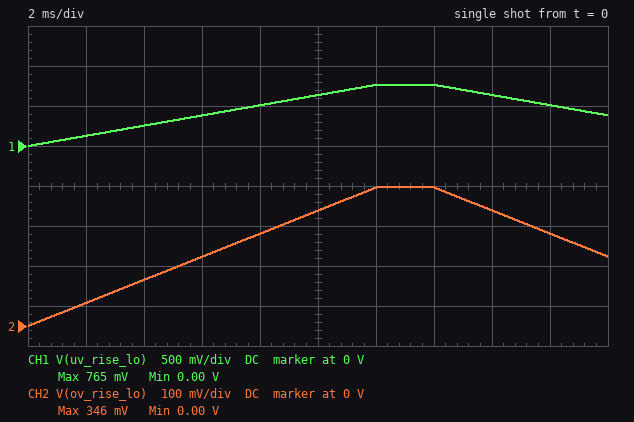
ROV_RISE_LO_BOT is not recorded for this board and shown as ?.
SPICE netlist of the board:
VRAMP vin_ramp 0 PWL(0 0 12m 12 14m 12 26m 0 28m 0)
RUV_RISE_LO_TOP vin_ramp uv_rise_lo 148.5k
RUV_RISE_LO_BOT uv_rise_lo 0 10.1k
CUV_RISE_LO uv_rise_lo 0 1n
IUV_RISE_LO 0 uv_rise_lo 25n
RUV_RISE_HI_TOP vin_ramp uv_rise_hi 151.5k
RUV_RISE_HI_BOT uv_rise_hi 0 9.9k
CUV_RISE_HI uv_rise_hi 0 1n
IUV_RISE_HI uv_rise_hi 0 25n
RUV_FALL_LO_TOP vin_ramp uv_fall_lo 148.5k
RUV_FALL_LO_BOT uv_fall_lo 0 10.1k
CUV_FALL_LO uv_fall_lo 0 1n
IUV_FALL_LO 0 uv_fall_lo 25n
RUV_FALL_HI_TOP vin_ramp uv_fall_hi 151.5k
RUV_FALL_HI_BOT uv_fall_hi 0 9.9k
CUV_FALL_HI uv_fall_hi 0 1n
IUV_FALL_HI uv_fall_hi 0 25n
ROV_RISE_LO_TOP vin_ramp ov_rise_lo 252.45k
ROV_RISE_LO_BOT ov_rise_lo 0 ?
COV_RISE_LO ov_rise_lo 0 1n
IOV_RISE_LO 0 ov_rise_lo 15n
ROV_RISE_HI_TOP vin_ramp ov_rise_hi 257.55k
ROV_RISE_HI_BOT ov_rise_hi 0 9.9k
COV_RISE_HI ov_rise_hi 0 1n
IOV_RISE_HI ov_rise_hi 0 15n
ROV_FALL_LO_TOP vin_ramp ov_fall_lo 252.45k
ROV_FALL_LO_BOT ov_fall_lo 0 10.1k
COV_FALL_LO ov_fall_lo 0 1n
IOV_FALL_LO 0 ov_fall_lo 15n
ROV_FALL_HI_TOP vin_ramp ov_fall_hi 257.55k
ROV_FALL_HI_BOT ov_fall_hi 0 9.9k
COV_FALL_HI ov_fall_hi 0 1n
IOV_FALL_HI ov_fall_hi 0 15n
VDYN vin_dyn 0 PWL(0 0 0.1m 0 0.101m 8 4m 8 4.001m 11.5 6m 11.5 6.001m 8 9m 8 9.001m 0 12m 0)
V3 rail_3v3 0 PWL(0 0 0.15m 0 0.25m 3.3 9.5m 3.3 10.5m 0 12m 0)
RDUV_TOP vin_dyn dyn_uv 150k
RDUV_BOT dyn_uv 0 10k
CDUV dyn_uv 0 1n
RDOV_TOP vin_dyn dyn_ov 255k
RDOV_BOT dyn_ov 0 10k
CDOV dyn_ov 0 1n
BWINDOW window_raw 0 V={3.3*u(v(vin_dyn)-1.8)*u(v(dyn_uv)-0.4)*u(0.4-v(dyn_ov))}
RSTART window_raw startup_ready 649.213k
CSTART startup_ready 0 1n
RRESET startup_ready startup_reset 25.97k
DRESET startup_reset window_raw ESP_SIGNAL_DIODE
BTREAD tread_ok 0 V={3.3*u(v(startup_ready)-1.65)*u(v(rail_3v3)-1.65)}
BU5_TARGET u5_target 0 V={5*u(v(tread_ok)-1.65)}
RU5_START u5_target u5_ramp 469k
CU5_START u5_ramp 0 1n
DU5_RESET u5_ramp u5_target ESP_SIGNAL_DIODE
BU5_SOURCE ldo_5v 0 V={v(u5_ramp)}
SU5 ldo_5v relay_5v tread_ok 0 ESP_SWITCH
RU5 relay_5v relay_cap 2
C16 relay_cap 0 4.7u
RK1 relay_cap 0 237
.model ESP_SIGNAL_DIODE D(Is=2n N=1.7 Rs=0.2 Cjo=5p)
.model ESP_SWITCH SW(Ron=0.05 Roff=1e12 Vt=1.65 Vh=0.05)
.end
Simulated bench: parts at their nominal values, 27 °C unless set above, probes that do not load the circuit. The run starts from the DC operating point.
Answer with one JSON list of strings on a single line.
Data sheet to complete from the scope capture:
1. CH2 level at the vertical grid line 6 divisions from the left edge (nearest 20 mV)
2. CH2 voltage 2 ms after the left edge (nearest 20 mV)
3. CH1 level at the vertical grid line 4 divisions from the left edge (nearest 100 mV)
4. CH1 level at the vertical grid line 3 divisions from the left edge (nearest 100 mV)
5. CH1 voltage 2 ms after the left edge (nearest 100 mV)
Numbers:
["340 mV", "60 mV", "500 mV", "400 mV", "100 mV"]
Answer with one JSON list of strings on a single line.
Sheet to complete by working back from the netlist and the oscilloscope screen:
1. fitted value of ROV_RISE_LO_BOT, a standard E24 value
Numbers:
["7.5 kΩ"]
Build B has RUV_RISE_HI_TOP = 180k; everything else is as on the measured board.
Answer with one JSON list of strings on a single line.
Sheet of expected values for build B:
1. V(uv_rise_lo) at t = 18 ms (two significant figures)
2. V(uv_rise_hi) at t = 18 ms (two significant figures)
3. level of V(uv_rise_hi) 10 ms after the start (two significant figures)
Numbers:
["510 mV", "420 mV", "520 mV"]
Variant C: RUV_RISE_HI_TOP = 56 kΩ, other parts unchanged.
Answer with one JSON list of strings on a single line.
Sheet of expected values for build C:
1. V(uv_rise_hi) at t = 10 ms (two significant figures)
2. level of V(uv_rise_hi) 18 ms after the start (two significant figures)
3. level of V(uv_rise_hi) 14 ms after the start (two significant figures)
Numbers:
["1.5 V", "1.2 V", "1.8 V"]
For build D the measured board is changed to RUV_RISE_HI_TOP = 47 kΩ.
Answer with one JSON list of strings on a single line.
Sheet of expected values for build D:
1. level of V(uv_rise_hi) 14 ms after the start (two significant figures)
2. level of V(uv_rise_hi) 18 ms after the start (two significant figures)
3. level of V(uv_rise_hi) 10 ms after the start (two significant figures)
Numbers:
["2.1 V", "1.4 V", "1.7 V"]
